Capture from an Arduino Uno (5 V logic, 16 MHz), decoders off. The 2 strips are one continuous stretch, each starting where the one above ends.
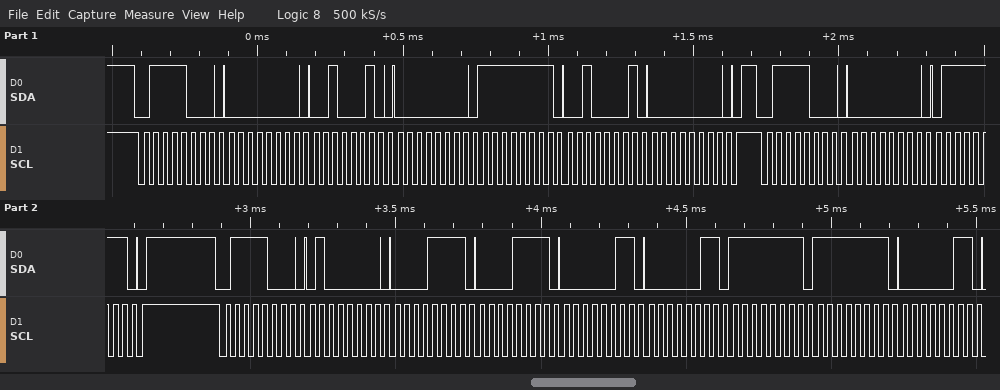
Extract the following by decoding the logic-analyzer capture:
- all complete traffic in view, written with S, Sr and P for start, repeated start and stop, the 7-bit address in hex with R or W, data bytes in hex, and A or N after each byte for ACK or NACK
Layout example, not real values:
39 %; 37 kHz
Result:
S 3CW A 00 A 22 A 00 A FF A 21 A 00 A P S 3CW A 00 A 7F A P S 3CW A 40 A 0F A 0F A 03 A 03 A FF A FF A 03 A
